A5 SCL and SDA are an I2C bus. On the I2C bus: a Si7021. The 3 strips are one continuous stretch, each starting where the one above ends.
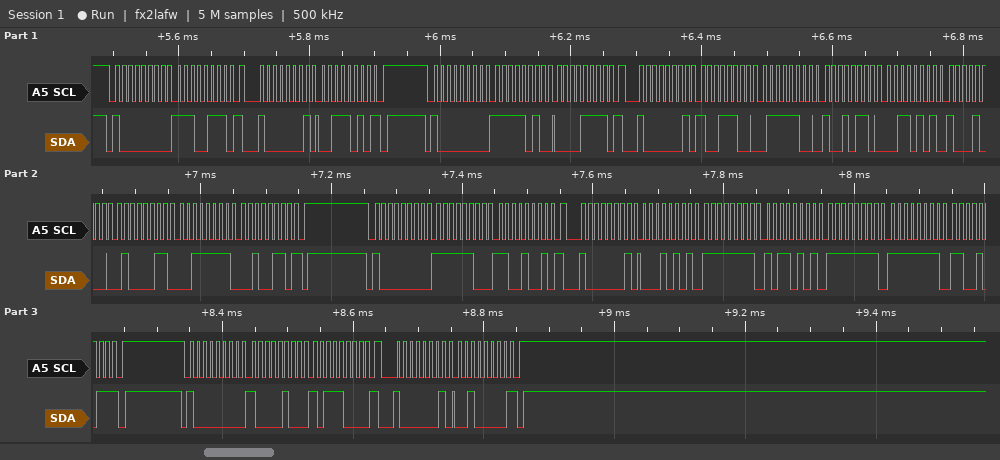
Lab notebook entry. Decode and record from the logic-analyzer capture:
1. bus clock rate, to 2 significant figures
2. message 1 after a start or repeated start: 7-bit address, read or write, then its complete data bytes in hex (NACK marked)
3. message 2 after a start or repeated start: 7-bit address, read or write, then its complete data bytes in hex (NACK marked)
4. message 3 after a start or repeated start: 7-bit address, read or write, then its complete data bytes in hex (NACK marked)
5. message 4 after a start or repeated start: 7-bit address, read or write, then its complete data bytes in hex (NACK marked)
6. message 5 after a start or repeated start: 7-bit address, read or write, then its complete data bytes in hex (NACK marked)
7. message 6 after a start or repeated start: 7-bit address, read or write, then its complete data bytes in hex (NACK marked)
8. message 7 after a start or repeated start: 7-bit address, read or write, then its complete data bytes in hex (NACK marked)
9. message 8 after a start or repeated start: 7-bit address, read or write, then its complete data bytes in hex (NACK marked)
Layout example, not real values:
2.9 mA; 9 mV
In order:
100 kHz; 0x40 write: E7; 0x40 read: 3A NACK; 0x40 write: FA 0F; 0x40 read: 9C 7C 96 35 88 43 3F 26 NACK; 0x40 write: FC C9; 0x40 read: 15 FF B5 FF FF CB NACK; 0x40 write: 84 B8; 0x40 read: 20 NACK
